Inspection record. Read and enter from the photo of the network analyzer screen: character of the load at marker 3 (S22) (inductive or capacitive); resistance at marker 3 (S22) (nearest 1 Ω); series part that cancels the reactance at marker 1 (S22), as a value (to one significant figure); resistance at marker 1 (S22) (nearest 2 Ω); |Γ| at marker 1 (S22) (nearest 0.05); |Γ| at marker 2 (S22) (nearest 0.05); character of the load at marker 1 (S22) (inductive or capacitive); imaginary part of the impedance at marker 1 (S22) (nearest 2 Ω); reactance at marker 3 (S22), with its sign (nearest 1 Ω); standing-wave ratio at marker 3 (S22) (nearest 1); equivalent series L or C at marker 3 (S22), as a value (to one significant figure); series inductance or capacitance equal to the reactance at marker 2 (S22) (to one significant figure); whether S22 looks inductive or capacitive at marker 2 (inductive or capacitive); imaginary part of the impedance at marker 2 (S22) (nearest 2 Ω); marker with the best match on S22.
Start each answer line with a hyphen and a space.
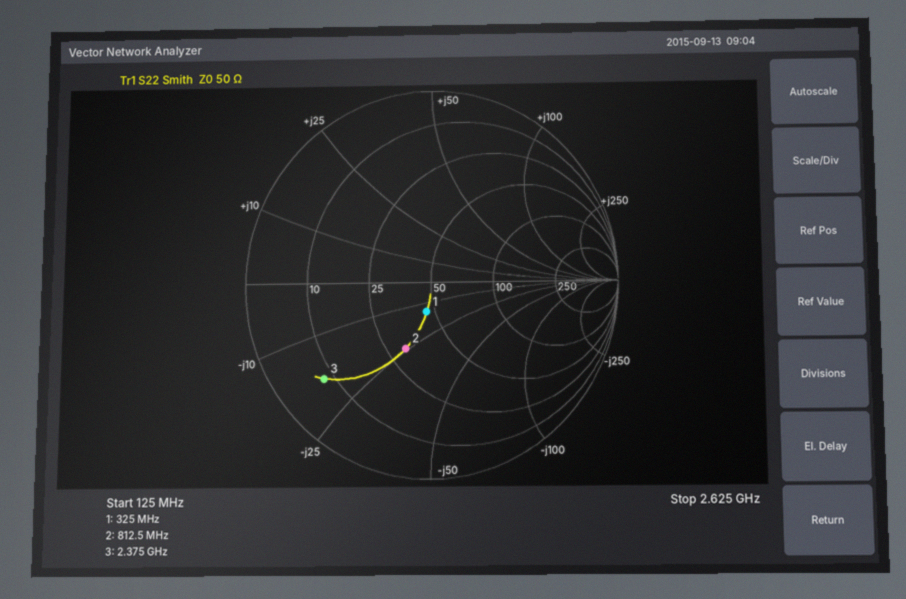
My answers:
- capacitive
- 8 Ω
- 7 nH
- 46 Ω
- 0.15
- 0.35
- capacitive
- -14 Ω
- -18 Ω
- 7
- 4 pF
- 8 pF
- capacitive
- -24 Ω
- marker 1
